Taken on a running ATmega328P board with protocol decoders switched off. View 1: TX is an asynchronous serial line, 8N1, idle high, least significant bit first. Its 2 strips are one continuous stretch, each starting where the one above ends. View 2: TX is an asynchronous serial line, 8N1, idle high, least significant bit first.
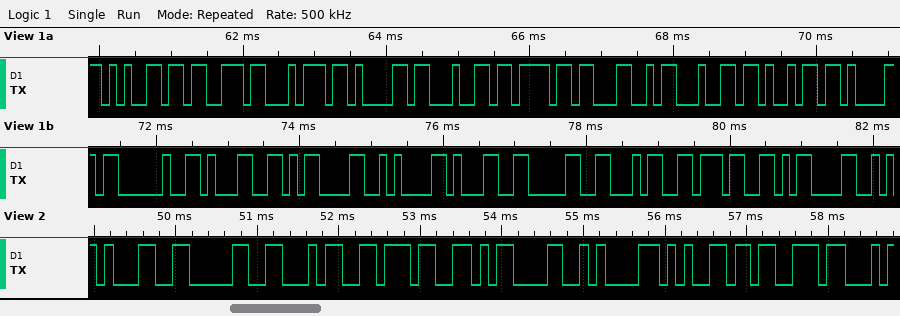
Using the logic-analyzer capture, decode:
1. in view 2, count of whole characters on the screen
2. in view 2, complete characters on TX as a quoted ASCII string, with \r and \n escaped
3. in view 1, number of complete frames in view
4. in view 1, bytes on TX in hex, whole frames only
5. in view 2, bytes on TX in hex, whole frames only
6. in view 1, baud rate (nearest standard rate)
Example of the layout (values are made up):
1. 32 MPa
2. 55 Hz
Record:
1. 8
2. "1047\r\nes"
3. 19
4. 65 73 74 61 64 6F 4C 64 69 61 20 31 0D 0A 31 30 34 37 0D
5. 31 30 34 37 0D 0A 65 73
6. 9600 baud
